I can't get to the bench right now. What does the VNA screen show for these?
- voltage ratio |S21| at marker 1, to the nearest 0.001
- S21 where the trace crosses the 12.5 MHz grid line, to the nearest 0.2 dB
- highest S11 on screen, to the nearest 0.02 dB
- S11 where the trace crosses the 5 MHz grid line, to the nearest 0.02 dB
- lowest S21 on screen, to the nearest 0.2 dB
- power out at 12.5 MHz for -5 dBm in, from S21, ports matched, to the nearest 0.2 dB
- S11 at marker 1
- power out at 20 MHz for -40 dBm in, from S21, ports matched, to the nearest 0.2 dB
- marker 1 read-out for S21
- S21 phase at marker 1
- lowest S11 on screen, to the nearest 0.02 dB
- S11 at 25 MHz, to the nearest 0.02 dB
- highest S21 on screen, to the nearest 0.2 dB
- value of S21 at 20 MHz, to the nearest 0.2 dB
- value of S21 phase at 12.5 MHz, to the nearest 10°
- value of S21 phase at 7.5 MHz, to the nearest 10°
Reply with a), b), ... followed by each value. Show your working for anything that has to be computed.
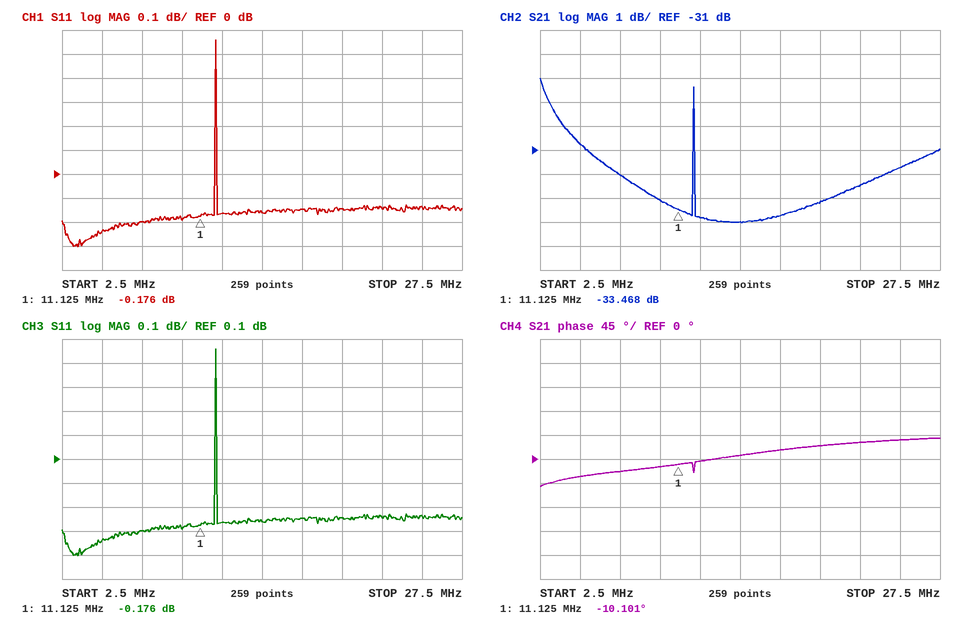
a) 10^(-33.468/20) ≈ 0.021
b) -33.8 dB
c) 0.56 dB
d) -0.24 dB
e) -34.0 dB
f) -5 dBm + (-33.8 dB) = -38.8 dBm
g) -0.176 dB
h) -40 dBm + (-33.2 dB) = -73.2 dBm
i) -33.468 dB
j) -10.101°
k) -0.30 dB
l) -0.14 dB
m) -28.0 dB
n) -33.2 dB
o) 0°
p) -20°
